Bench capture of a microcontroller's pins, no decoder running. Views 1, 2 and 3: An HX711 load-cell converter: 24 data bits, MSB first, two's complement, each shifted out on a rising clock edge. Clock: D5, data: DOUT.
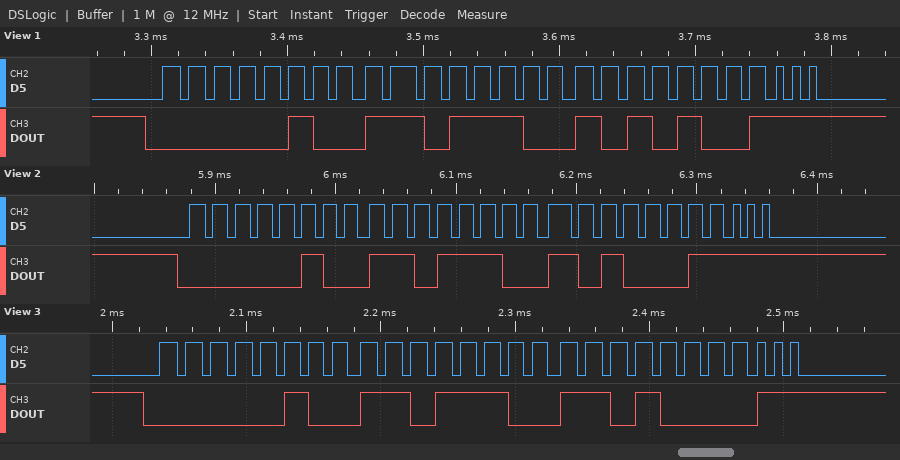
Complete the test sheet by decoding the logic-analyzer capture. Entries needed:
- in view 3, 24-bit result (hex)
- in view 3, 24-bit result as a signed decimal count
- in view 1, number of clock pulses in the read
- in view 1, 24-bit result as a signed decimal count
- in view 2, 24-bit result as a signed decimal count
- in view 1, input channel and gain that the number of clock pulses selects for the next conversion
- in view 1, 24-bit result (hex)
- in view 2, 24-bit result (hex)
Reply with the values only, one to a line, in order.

0x04DCD0
318672
27
318633
318627
channel A, gain 64
0x04DCA9
0x04DCA3
